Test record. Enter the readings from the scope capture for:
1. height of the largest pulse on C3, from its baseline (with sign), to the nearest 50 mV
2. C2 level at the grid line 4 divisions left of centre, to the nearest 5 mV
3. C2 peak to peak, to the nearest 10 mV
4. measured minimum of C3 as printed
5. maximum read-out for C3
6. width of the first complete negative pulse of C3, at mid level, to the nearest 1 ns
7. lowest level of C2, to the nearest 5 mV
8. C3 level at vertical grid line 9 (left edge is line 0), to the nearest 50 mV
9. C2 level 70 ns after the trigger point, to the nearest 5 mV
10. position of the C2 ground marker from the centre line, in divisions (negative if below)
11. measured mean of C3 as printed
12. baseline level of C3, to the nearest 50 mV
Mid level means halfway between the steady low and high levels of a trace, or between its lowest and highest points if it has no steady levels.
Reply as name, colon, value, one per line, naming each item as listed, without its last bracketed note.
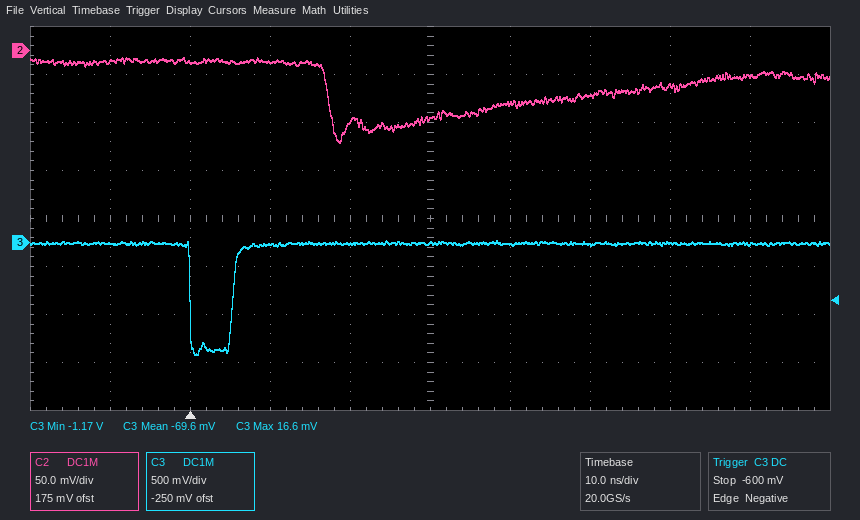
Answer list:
height of the largest pulse on C3, from its baseline (with sign), to the nearest 50 mV: -1.15 V
C2 level at the grid line 4 divisions left of centre, to the nearest 5 mV: -10 mV
C2 peak to peak, to the nearest 10 mV: 90 mV
measured minimum of C3 as printed: -1.17 V
maximum read-out for C3: 16.6 mV
width of the first complete negative pulse of C3, at mid level, to the nearest 1 ns: 5 ns
lowest level of C2, to the nearest 5 mV: -95 mV
C3 level at vertical grid line 9 (left edge is line 0), to the nearest 50 mV: 0 mV
C2 level 70 ns after the trigger point, to the nearest 5 mV: -25 mV
position of the C2 ground marker from the centre line, in divisions: +3.5 div
measured mean of C3 as printed: -69.6 mV
baseline level of C3, to the nearest 50 mV: 0 mV
